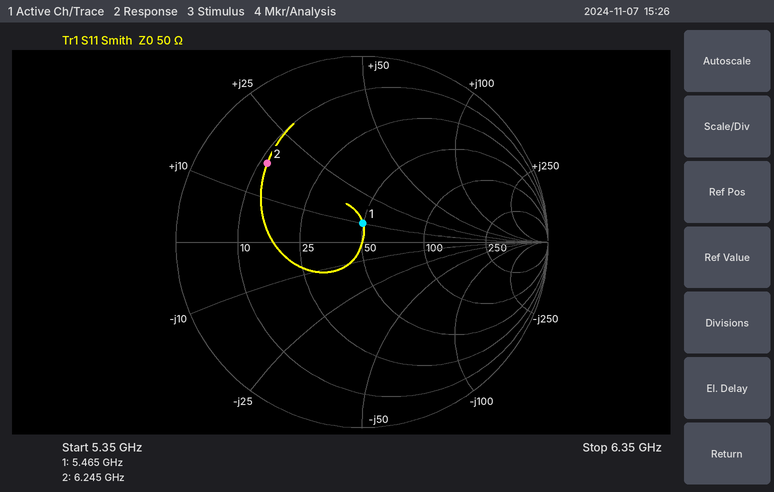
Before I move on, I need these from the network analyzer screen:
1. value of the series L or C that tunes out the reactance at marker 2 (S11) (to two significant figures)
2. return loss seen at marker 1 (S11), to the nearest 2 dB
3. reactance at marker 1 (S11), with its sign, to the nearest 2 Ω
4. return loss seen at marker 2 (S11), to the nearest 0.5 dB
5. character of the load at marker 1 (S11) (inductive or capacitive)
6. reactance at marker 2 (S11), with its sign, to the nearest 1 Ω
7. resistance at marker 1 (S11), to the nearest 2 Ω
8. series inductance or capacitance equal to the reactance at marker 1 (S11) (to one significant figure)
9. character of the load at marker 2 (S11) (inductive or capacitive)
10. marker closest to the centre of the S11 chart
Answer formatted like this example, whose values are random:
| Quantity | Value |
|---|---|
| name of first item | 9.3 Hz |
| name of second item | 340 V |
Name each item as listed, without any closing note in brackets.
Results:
| Quantity | Value |
|---|---|
| value of the series L or C that tunes out the reactance at marker 2 (S11) | 1.5 pF |
| return loss seen at marker 1 (S11), to the nearest 2 dB | 20 dB |
| reactance at marker 1 (S11), with its sign, to the nearest 2 Ω | +10 Ω |
| return loss seen at marker 2 (S11), to the nearest 0.5 dB | 3.5 dB |
| character of the load at marker 1 (S11) | inductive |
| reactance at marker 2 (S11), with its sign, to the nearest 1 Ω | +17 Ω |
| resistance at marker 1 (S11), to the nearest 2 Ω | 50 Ω |
| series inductance or capacitance equal to the reactance at marker 1 (S11) | 300 pH |
| character of the load at marker 2 (S11) | inductive |
| marker closest to the centre of the S11 chart | marker 1 |
